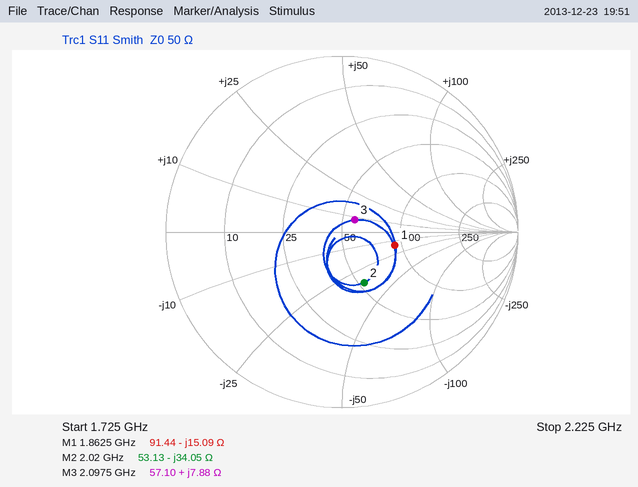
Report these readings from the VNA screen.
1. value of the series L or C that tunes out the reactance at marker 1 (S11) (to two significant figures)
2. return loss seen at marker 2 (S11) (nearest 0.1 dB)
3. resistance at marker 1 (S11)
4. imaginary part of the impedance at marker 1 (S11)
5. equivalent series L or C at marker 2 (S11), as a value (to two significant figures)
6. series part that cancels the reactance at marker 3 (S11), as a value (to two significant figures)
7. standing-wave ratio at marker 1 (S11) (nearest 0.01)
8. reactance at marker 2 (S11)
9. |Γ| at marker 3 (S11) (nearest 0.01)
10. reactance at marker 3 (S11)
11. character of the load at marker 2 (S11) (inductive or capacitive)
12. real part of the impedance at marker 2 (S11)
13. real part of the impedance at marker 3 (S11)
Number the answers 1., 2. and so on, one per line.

1. 1.3 nH
2. 10.0 dB
3. 91.44 Ω
4. -15.09 Ω
5. 2.3 pF
6. 9.6 pF
7. 1.90
8. -34.05 Ω
9. 0.10
10. +7.88 Ω
11. capacitive
12. 53.13 Ω
13. 57.10 Ω
